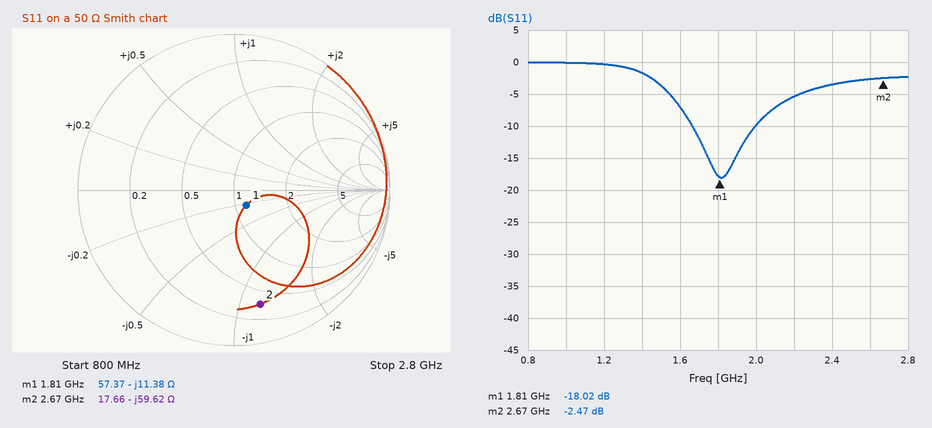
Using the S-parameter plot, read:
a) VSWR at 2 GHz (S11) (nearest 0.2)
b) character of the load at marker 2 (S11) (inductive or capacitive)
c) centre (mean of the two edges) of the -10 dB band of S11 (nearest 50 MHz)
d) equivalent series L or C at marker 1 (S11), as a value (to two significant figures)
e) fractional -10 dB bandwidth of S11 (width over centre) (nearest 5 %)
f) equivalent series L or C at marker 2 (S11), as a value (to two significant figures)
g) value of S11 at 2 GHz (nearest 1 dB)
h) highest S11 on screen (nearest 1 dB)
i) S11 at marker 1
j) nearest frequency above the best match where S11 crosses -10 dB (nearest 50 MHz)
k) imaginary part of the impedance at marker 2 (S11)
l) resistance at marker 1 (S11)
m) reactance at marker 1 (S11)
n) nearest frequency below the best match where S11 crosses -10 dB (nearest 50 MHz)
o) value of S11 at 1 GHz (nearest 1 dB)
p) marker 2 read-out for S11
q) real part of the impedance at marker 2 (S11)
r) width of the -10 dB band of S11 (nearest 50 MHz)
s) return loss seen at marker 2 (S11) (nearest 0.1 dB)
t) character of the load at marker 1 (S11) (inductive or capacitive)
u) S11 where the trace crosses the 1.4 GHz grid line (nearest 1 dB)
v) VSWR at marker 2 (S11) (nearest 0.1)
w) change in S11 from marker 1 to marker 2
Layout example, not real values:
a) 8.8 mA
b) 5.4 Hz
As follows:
a) 2.0
b) capacitive
c) 1.85 GHz
d) 7.7 pF
e) 20 %
f) 1.00 pF
g) -10 dB
h) 0 dB
i) -18.02 dB
j) 2.00 GHz
k) -59.62 Ω
l) 57.37 Ω
m) -11.38 Ω
n) 1.65 GHz
o) 0 dB
p) -2.47 dB
q) 17.66 Ω
r) 350 MHz
s) 2.5 dB
t) capacitive
u) -2 dB
v) 7.1
w) 15.55 dB
